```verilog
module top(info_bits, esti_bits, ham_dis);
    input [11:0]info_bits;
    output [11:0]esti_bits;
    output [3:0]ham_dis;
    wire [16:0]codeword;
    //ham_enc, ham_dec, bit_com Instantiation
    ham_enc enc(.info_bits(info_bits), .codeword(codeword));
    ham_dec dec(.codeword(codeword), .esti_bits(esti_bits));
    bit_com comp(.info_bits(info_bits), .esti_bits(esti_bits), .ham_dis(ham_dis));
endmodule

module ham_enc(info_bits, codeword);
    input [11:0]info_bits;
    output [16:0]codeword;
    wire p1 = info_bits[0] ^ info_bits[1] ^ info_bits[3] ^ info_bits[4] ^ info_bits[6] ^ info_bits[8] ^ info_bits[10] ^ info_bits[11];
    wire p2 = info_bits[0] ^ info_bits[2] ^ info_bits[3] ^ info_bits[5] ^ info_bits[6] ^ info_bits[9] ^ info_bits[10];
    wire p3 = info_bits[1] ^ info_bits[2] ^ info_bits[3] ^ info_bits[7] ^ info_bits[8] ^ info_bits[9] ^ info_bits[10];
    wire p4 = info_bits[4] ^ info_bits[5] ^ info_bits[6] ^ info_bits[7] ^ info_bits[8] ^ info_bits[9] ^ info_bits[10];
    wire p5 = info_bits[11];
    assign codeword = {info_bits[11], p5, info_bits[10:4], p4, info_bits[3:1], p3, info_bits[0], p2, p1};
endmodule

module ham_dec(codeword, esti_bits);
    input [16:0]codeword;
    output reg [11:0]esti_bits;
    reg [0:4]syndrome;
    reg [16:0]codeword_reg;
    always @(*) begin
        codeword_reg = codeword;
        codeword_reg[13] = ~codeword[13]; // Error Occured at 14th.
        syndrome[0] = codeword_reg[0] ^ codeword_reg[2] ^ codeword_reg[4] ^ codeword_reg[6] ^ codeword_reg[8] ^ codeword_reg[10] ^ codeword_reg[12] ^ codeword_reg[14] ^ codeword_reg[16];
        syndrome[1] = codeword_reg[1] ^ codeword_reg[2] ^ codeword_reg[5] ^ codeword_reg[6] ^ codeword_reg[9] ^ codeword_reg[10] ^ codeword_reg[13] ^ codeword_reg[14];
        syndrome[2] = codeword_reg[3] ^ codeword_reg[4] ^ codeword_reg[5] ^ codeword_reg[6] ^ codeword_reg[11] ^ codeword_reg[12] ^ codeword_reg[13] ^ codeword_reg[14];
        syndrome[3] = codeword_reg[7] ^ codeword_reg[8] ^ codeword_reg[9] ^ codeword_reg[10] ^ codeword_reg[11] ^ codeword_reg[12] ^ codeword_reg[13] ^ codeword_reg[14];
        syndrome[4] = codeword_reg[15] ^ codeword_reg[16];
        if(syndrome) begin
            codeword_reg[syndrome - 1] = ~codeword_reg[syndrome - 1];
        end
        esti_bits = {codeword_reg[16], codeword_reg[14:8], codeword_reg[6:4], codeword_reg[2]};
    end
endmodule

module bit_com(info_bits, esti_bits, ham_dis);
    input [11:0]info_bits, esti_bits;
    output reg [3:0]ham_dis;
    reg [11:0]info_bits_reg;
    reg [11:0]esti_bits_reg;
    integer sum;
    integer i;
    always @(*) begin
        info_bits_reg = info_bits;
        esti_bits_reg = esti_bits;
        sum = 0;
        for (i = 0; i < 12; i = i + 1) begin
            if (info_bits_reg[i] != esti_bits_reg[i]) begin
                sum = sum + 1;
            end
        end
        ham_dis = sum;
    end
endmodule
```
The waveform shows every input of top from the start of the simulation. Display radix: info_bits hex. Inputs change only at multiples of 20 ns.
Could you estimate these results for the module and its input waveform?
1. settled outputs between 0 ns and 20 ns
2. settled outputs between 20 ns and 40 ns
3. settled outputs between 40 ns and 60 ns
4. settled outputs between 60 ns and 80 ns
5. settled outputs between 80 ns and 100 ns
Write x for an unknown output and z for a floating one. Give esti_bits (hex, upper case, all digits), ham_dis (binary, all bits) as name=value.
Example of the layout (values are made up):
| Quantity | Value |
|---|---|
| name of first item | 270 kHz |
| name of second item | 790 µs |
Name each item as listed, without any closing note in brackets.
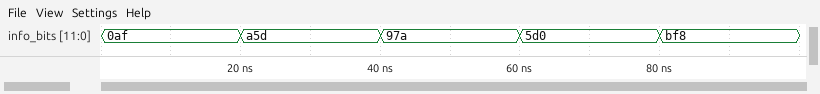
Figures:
| Quantity | Value |
|---|---|
| settled outputs between 0 ns and 20 ns | esti_bits=0AF, ham_dis=0000 |
| settled outputs between 20 ns and 40 ns | esti_bits=A5D, ham_dis=0000 |
| settled outputs between 40 ns and 60 ns | esti_bits=97A, ham_dis=0000 |
| settled outputs between 60 ns and 80 ns | esti_bits=5D0, ham_dis=0000 |
| settled outputs between 80 ns and 100 ns | esti_bits=BF8, ham_dis=0000 |
